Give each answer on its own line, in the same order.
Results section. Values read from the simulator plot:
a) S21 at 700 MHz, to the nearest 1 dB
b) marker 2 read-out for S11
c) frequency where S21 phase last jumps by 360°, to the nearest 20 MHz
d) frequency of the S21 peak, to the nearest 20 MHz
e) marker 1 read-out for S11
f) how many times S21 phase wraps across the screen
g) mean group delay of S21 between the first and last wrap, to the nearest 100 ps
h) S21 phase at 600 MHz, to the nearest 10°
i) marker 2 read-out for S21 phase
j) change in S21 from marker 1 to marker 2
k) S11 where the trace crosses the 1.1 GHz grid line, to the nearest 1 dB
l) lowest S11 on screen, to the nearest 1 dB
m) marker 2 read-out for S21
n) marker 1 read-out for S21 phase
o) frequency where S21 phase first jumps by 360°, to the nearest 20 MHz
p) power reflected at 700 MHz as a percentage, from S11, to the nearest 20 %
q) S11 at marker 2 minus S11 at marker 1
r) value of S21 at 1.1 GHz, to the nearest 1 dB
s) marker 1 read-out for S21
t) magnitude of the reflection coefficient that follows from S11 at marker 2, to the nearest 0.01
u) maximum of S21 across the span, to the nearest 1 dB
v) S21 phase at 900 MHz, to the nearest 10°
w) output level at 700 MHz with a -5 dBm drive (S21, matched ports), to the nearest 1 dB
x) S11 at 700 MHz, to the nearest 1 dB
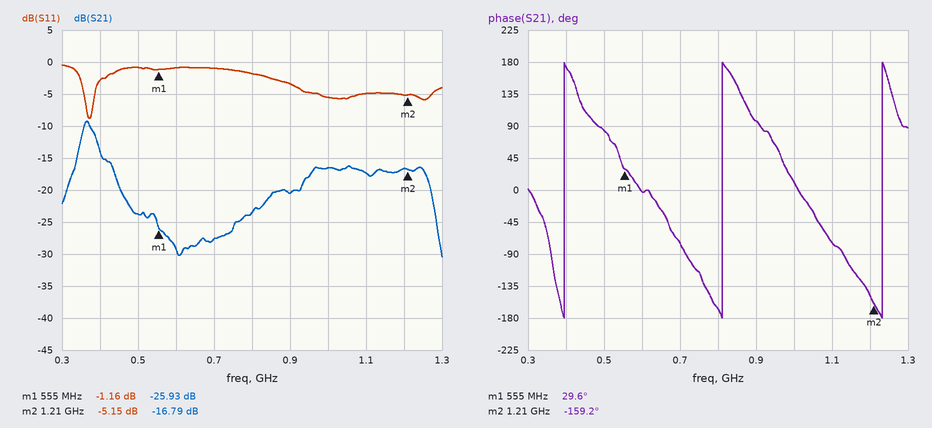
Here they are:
-28 dB
-5.15 dB
1.24 GHz
360 MHz
-1.16 dB
3
2.4 ns
0°
-159.2°
9.14 dB
-5 dB
-9 dB
-16.79 dB
29.6°
400 MHz
80 %
-3.99 dB
-17 dB
-25.93 dB
0.55
-9 dB
100°
-33 dBm
-1 dB
